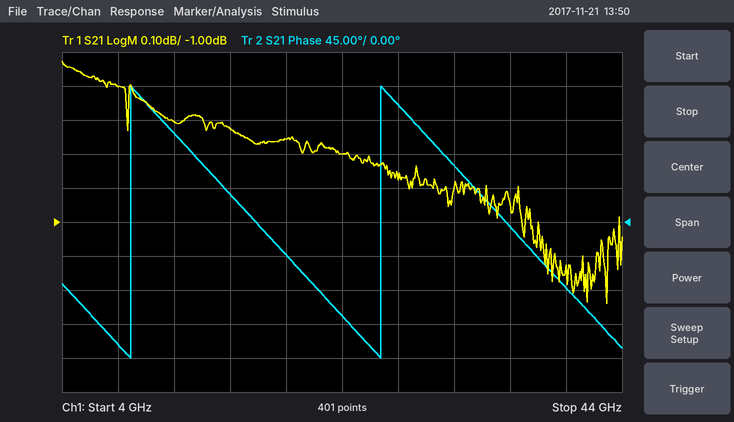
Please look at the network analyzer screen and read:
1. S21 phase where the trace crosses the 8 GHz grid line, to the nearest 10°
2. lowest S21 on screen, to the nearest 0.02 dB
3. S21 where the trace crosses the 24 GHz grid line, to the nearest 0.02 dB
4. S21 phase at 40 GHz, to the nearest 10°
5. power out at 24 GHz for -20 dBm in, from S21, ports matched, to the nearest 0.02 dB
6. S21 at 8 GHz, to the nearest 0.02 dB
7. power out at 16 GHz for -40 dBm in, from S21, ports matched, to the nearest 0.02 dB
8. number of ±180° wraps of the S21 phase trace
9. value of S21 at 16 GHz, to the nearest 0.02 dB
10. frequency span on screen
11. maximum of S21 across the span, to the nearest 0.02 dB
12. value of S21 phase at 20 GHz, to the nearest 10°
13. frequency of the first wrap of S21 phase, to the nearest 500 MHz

-160°
-1.24 dB
-0.80 dB
-90°
-20.80 dBm
-0.60 dB
-40.72 dBm
2
-0.72 dB
40 GHz
-0.52 dB
-40°
9.0 GHz
